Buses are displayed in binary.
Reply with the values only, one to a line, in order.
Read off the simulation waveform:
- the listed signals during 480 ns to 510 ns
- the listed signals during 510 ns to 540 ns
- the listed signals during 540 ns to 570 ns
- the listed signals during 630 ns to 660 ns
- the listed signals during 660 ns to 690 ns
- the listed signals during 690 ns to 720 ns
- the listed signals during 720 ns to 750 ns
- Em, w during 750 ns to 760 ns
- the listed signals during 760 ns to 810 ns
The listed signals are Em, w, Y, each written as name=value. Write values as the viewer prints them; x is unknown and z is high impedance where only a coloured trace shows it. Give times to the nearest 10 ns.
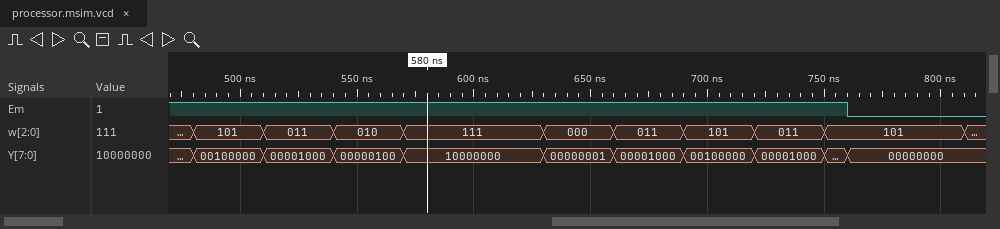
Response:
Em=1, w=101, Y=00100000
Em=1, w=011, Y=00001000
Em=1, w=010, Y=00000100
Em=1, w=000, Y=00000001
Em=1, w=011, Y=00001000
Em=1, w=101, Y=00100000
Em=1, w=011, Y=00001000
Em=1, w=101
Em=0, w=101, Y=00000000
